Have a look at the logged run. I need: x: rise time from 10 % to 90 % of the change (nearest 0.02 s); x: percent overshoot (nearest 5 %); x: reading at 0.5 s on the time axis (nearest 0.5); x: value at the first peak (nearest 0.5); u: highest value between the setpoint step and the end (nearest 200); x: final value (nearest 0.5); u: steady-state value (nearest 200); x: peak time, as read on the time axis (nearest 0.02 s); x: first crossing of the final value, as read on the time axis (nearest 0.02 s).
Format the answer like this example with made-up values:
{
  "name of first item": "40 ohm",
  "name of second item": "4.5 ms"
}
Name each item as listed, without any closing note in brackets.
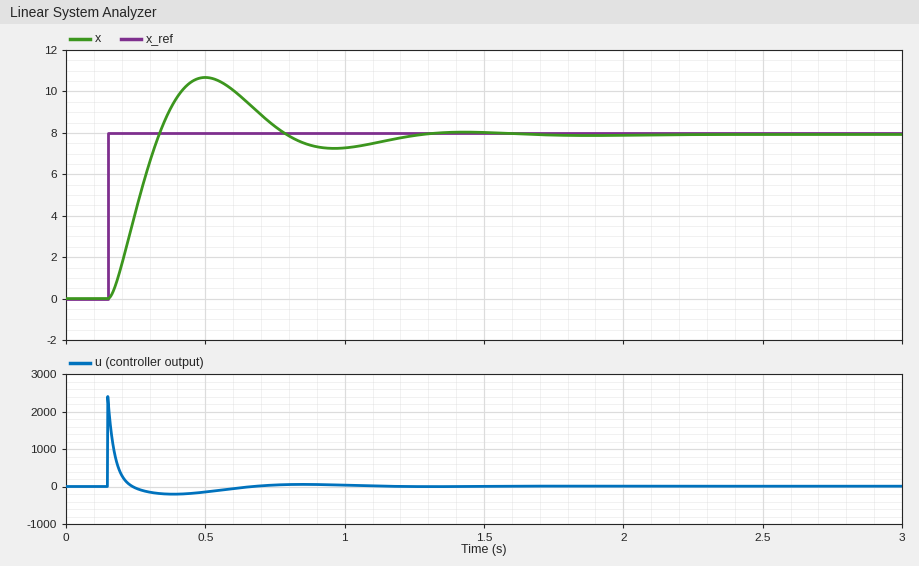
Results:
{
  "x: rise time from 10 % to 90 % of the change": "0.14 s",
  "x: percent overshoot": "35 %",
  "x: reading at 0.5 s on the time axis": "10.5",
  "x: value at the first peak": "10.5",
  "u: highest value between the setpoint step and the end": "2400",
  "x: final value": "8.0",
  "u: steady-state value": "0",
  "x: peak time, as read on the time axis": "0.50 s",
  "x: first crossing of the final value, as read on the time axis": "0.34 s"
}
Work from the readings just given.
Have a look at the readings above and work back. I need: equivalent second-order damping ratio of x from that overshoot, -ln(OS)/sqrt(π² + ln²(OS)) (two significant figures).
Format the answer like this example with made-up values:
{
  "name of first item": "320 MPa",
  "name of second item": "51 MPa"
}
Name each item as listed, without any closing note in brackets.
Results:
{
  "equivalent second-order damping ratio of x from that overshoot, -ln(OS)/sqrt(π² + ln²(OS))": "0.32"
}
